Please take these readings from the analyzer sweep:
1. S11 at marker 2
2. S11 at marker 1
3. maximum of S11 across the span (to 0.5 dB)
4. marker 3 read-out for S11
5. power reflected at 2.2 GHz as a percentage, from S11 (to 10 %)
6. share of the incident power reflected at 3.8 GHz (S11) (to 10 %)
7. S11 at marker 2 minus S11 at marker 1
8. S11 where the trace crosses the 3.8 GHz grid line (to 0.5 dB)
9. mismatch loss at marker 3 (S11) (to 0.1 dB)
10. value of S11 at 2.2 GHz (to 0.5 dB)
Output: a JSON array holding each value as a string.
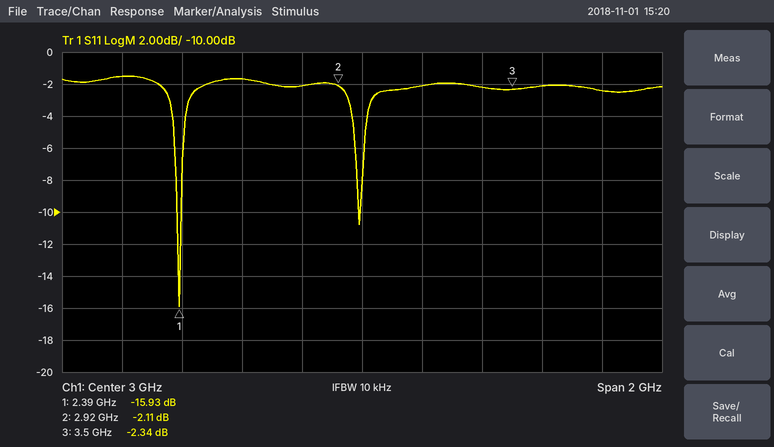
["-2.11 dB", "-15.93 dB", "-1.5 dB", "-2.34 dB", "70 %", "60 %", "13.82 dB", "-2.5 dB", "3.8 dB", "-1.5 dB"]
